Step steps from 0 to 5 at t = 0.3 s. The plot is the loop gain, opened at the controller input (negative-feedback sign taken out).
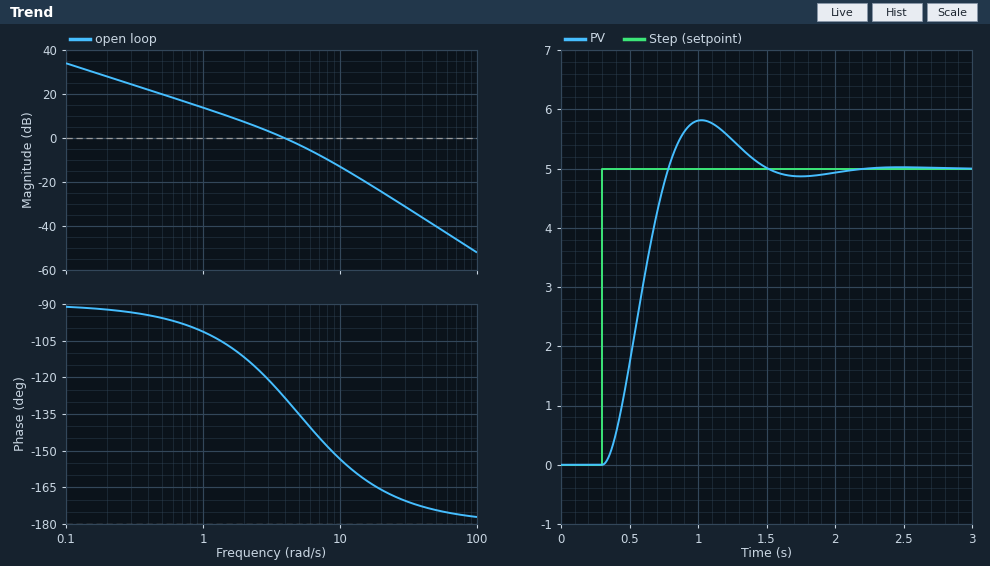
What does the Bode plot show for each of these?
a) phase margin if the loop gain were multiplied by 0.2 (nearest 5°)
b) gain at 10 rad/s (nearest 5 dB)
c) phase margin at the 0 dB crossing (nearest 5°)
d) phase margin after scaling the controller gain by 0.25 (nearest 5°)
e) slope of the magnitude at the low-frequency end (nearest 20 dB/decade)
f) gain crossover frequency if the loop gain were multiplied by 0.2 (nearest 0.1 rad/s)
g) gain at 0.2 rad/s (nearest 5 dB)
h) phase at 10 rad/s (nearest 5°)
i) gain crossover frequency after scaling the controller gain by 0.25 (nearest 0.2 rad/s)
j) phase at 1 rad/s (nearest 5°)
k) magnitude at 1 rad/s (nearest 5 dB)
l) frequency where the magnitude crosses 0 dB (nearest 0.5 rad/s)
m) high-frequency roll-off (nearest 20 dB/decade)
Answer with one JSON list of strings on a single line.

["80°", "-15 dB", "50°", "75°", "-20 dB/decade", "1.0 rad/s", "30 dB", "-155°", "1.2 rad/s", "-100°", "15 dB", "4.0 rad/s", "-40 dB/decade"]
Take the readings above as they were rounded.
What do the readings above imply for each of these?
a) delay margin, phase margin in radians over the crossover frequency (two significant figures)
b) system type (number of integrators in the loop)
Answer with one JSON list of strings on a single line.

["0.22 s", "1"]
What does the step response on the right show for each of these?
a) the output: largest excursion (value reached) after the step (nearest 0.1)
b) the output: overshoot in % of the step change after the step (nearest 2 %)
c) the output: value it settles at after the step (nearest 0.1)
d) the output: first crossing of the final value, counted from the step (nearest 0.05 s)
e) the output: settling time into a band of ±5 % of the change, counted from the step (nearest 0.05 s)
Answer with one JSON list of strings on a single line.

["5.8", "16 %", "5.0", "0.50 s", "1.05 s"]
